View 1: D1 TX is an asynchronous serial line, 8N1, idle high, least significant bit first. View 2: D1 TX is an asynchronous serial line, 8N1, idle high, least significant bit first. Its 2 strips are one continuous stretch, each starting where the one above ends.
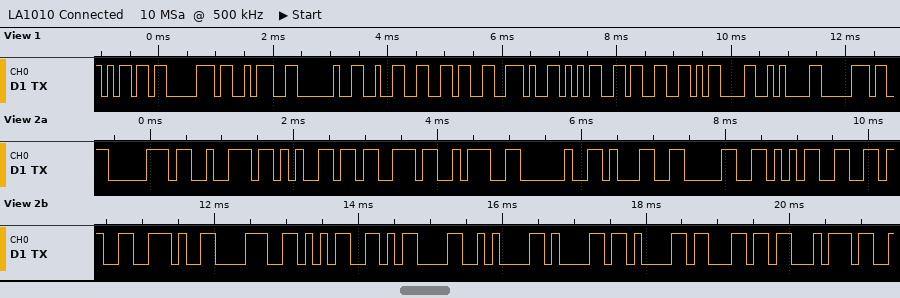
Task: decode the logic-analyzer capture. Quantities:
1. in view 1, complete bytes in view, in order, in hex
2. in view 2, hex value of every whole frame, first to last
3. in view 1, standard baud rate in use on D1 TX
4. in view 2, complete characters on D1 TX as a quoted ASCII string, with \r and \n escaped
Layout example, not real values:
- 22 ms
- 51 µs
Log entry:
- 6D 70 3A 20 32 36 2E 35 33 0D 0A 70
- 70 72 65 73 3A 20 31 30 35 36 2E 38 35 0D 0A 61 61 6C 74
- 9600 baud
- "pres: 1056.85\r\naalt"
